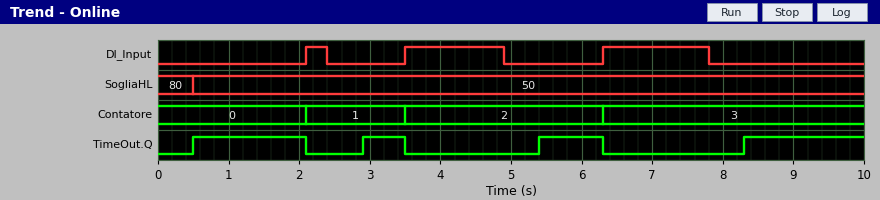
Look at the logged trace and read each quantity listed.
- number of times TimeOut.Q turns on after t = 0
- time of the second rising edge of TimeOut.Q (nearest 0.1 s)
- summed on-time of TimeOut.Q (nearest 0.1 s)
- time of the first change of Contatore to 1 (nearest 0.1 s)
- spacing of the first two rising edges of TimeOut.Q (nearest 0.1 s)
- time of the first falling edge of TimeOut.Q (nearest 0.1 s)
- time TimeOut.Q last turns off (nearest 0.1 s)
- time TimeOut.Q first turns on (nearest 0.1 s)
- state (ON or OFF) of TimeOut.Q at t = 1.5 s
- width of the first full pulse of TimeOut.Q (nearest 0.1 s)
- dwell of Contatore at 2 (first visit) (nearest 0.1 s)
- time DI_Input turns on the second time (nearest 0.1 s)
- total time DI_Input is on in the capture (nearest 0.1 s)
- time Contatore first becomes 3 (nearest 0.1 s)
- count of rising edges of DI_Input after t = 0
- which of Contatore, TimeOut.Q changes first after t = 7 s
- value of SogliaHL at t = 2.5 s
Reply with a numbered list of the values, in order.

1. 4
2. 2.9 s
3. 4.8 s
4. 2.1 s
5. 2.4 s
6. 2.1 s
7. 6.3 s
8. 0.5 s
9. ON
10. 1.6 s
11. 2.8 s
12. 3.5 s
13. 3.2 s
14. 6.3 s
15. 3
16. TimeOut.Q
17. 50
